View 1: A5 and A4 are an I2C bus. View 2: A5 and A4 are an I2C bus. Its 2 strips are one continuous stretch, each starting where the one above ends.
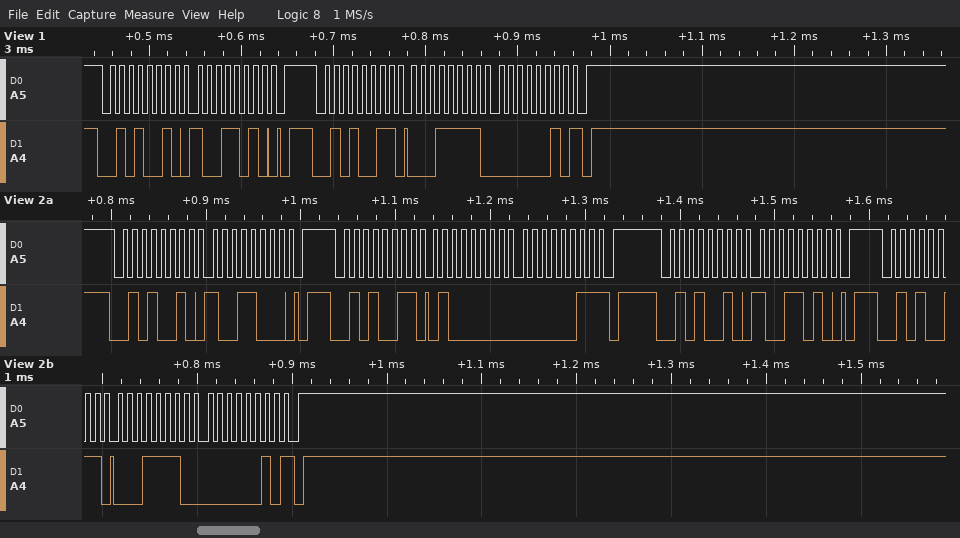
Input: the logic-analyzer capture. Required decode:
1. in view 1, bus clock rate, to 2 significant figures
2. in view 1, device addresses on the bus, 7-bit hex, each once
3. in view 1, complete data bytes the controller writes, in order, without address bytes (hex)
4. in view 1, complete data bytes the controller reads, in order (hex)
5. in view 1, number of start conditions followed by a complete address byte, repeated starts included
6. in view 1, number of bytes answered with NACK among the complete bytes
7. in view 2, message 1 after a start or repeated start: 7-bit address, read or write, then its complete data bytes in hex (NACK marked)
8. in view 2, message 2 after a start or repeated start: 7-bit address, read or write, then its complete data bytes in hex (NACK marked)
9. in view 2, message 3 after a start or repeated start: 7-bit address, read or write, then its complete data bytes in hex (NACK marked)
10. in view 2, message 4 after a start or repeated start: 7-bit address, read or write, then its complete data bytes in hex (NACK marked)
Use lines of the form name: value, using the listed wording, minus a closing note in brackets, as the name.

in view 1, bus clock rate, to 2 significant figures: 100 kHz
in view 1, device addresses on the bus, 7-bit hex, each once: 0x29
in view 1, complete data bytes the controller writes, in order, without address bytes: 9A
in view 1, complete data bytes the controller reads, in order: 1F 02
in view 1, number of start conditions followed by a complete address byte, repeated starts included: 2
in view 1, number of bytes answered with NACK among the complete bytes: 1
in view 2, message 1 after a start or repeated start: 7-bit address, read or write, then its complete data bytes in hex: 0x29 write: 98
in view 2, message 2 after a start or repeated start: 7-bit address, read or write, then its complete data bytes in hex: 0x29 read: 40 03 NACK
in view 2, message 3 after a start or repeated start: 7-bit address, read or write, then its complete data bytes in hex: 0x29 write: 9A
in view 2, message 4 after a start or repeated start: 7-bit address, read or write, then its complete data bytes in hex: 0x29 read: 1E 02 NACK
